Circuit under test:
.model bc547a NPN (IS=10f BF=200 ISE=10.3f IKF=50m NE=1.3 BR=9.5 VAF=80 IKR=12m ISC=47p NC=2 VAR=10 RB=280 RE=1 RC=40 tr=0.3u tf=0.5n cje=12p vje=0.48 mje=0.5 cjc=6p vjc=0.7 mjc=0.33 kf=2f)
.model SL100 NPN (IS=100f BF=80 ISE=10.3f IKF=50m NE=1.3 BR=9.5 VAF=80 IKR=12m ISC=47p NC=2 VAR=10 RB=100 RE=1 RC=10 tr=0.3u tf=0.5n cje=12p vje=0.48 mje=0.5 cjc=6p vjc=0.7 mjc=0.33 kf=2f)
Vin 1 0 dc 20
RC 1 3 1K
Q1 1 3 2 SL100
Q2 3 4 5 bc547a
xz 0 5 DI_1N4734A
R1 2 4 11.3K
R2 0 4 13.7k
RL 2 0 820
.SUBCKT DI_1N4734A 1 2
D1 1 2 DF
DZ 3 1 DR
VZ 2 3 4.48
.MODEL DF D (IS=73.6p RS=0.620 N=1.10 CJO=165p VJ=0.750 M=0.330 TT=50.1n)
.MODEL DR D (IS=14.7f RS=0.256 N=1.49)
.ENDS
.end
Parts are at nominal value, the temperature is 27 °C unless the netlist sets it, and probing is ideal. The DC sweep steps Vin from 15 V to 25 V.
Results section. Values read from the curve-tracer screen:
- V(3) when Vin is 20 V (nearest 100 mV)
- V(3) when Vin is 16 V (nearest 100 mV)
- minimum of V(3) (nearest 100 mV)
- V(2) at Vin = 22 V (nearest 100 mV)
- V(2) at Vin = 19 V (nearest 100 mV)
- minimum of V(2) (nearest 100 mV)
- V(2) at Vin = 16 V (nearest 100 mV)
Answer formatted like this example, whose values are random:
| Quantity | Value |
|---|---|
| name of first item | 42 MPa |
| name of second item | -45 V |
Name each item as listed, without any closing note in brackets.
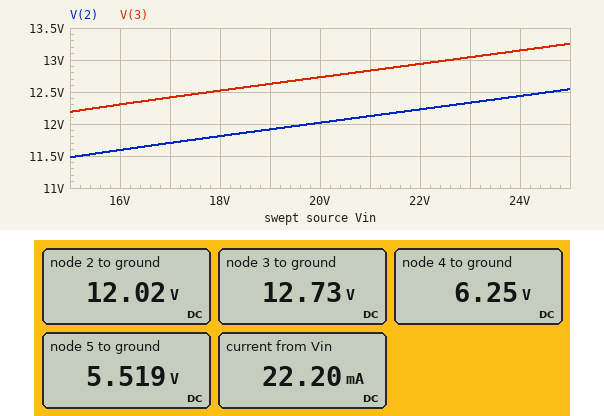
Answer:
| Quantity | Value |
|---|---|
| V(3) when Vin is 20 V | 12.7 V |
| V(3) when Vin is 16 V | 12.3 V |
| minimum of V(3) | 12.2 V |
| V(2) at Vin = 22 V | 12.2 V |
| V(2) at Vin = 19 V | 11.9 V |
| minimum of V(2) | 11.5 V |
| V(2) at Vin = 16 V | 11.6 V |
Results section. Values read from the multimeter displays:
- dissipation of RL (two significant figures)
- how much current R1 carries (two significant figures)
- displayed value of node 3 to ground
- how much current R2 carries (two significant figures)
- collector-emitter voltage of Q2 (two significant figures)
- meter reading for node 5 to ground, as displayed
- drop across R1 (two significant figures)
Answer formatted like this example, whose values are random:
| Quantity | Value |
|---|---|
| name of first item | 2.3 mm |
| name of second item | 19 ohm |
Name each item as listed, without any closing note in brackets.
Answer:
| Quantity | Value |
|---|---|
| dissipation of RL | 180 mW |
| how much current R1 carries | 510 µA |
| displayed value of node 3 to ground | 12.73 V |
| how much current R2 carries | 460 µA |
| collector-emitter voltage of Q2 | 7.2 V |
| meter reading for node 5 to ground, as displayed | 5.519 V |
| drop across R1 | 5.8 V |
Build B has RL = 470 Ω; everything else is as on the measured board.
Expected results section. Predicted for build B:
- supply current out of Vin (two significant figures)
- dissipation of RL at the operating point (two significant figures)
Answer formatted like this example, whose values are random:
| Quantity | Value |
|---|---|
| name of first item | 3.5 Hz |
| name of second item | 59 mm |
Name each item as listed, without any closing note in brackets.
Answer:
| Quantity | Value |
|---|---|
| supply current out of Vin | 33 mA |
| dissipation of RL at the operating point | 310 mW |
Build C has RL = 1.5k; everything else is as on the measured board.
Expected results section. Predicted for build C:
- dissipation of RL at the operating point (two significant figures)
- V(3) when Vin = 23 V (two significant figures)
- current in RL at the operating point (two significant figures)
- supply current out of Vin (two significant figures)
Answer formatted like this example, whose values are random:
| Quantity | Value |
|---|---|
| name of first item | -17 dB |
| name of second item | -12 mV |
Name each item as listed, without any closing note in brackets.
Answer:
| Quantity | Value |
|---|---|
| dissipation of RL at the operating point | 97 mW |
| V(3) when Vin = 23 V | 13 V |
| current in RL at the operating point | 8.0 mA |
| supply current out of Vin | 16 mA |
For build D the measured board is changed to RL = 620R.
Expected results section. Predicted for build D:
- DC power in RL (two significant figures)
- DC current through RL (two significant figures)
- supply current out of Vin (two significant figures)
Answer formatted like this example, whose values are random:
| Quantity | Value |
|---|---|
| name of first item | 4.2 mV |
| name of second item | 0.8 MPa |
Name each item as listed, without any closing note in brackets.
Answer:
| Quantity | Value |
|---|---|
| DC power in RL | 230 mW |
| DC current through RL | 19 mA |
| supply current out of Vin | 27 mA |
